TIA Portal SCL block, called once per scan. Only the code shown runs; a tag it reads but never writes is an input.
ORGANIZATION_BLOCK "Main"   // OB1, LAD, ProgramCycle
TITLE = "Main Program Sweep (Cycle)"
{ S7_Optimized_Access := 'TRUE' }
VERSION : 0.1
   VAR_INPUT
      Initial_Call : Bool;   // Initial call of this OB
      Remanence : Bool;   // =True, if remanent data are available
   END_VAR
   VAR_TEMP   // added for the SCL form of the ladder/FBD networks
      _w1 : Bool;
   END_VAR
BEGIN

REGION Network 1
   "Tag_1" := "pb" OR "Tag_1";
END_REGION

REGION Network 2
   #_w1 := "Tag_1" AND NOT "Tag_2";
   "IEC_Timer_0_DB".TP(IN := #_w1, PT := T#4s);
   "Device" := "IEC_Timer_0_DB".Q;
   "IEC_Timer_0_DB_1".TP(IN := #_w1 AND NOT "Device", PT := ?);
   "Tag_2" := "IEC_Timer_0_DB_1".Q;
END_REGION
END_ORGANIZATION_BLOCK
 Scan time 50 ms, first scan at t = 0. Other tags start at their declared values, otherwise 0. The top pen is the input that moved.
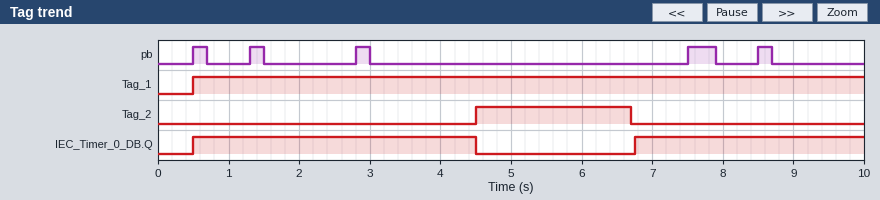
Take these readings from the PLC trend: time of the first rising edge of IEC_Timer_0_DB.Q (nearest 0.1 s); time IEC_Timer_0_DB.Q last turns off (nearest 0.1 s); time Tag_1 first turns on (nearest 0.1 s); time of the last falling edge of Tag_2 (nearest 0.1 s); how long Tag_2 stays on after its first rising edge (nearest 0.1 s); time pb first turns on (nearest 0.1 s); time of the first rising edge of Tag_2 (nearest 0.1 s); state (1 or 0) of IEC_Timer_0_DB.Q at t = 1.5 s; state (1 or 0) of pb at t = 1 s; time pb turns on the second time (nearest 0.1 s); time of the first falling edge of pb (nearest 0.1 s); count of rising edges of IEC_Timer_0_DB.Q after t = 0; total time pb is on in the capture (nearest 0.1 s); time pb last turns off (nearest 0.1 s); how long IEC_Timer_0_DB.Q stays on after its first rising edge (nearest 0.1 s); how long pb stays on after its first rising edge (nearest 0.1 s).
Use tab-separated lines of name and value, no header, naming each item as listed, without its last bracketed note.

time of the first rising edge of IEC_Timer_0_DB.Q	0.5 s
time IEC_Timer_0_DB.Q last turns off	4.5 s
time Tag_1 first turns on	0.5 s
time of the last falling edge of Tag_2	6.7 s
how long Tag_2 stays on after its first rising edge	2.2 s
time pb first turns on	0.5 s
time of the first rising edge of Tag_2	4.5 s
state (1 or 0) of IEC_Timer_0_DB.Q at t = 1.5 s	1
state (1 or 0) of pb at t = 1 s	0
time pb turns on the second time	1.3 s
time of the first falling edge of pb	0.7 s
count of rising edges of IEC_Timer_0_DB.Q after t = 0	2
total time pb is on in the capture	1.2 s
time pb last turns off	8.7 s
how long IEC_Timer_0_DB.Q stays on after its first rising edge	4.0 s
how long pb stays on after its first rising edge	0.2 s
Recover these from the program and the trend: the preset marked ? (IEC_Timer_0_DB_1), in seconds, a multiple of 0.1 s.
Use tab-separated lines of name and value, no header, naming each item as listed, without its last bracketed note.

the preset marked ? (IEC_Timer_0_DB_1), in seconds, a multiple of 0.1 s	2.2 s
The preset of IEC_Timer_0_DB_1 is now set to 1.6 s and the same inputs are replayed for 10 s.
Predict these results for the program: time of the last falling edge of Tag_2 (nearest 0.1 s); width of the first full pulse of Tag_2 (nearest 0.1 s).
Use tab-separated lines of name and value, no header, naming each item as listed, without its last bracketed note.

time of the last falling edge of Tag_2	6.1 s
width of the first full pulse of Tag_2	1.6 s
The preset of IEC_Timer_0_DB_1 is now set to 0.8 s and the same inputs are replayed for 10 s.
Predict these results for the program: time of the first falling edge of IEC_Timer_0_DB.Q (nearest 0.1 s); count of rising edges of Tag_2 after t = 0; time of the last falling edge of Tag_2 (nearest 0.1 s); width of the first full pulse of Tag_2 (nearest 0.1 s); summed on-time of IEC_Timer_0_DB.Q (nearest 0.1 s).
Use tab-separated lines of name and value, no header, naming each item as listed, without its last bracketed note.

time of the first falling edge of IEC_Timer_0_DB.Q	4.5 s
count of rising edges of Tag_2 after t = 0	2
time of the last falling edge of Tag_2	5.3 s
width of the first full pulse of Tag_2	0.8 s
summed on-time of IEC_Timer_0_DB.Q	8.0 s
